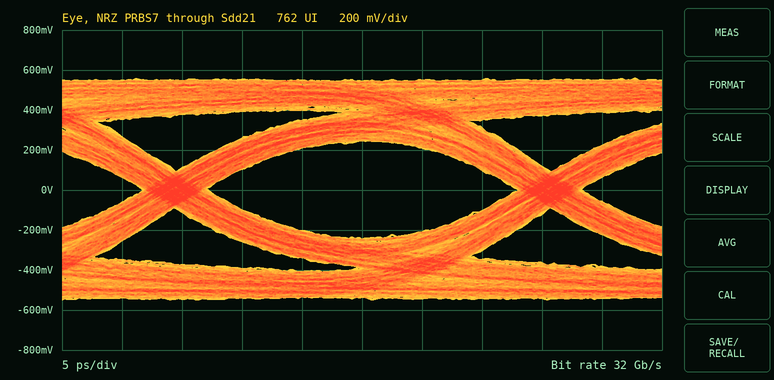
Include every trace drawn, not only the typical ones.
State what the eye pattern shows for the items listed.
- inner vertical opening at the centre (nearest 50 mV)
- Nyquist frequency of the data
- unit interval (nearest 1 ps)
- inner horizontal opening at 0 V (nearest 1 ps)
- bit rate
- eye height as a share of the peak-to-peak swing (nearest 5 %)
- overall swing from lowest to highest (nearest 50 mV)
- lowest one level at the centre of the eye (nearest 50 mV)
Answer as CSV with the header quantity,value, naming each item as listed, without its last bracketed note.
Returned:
quantity,value
inner vertical opening at the centre,500 mV
Nyquist frequency of the data,16 GHz
unit interval,31 ps
inner horizontal opening at 0 V,26 ps
bit rate,32 Gb/s
eye height as a share of the peak-to-peak swing,45 %
overall swing from lowest to highest,1.10 V
lowest one level at the centre of the eye,250 mV
